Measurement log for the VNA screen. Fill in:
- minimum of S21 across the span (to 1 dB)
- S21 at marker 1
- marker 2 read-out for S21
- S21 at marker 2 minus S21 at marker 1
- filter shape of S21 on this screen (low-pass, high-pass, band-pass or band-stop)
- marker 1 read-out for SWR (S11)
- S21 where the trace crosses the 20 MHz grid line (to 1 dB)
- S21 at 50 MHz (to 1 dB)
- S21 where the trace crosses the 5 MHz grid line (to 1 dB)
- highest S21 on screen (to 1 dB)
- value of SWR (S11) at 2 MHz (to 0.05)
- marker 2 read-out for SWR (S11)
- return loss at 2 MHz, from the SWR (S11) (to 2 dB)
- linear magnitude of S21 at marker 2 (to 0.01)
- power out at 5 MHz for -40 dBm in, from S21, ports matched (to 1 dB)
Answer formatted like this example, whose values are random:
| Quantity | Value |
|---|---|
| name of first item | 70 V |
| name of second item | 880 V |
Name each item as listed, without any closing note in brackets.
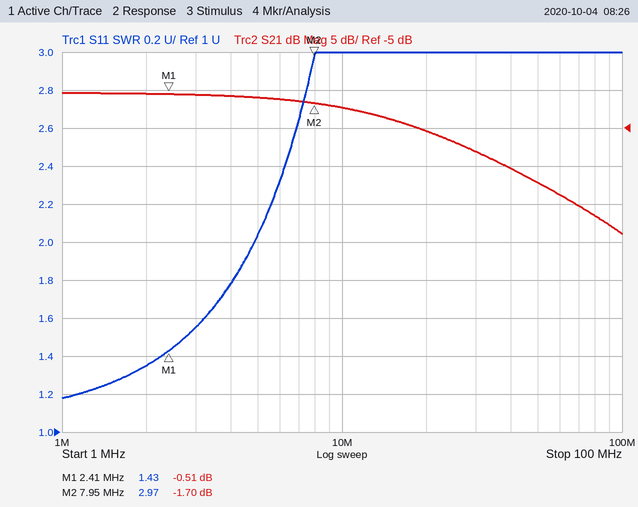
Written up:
| Quantity | Value |
|---|---|
| minimum of S21 across the span | -19 dB |
| S21 at marker 1 | -0.51 dB |
| marker 2 read-out for S21 | -1.70 dB |
| S21 at marker 2 minus S21 at marker 1 | -1.19 dB |
| filter shape of S21 on this screen | low-pass |
| marker 1 read-out for SWR | 1.43 |
| S21 where the trace crosses the 20 MHz grid line | -5 dB |
| S21 at 50 MHz | -12 dB |
| S21 where the trace crosses the 5 MHz grid line | -1 dB |
| highest S21 on screen | 0 dB |
| value of SWR (S11) at 2 MHz | 1.35 |
| marker 2 read-out for SWR | 2.97 |
| return loss at 2 MHz, from the SWR (S11) | 16 dB |
| linear magnitude of S21 at marker 2 | 0.82 |
| power out at 5 MHz for -40 dBm in, from S21, ports matched | -41 dBm |
